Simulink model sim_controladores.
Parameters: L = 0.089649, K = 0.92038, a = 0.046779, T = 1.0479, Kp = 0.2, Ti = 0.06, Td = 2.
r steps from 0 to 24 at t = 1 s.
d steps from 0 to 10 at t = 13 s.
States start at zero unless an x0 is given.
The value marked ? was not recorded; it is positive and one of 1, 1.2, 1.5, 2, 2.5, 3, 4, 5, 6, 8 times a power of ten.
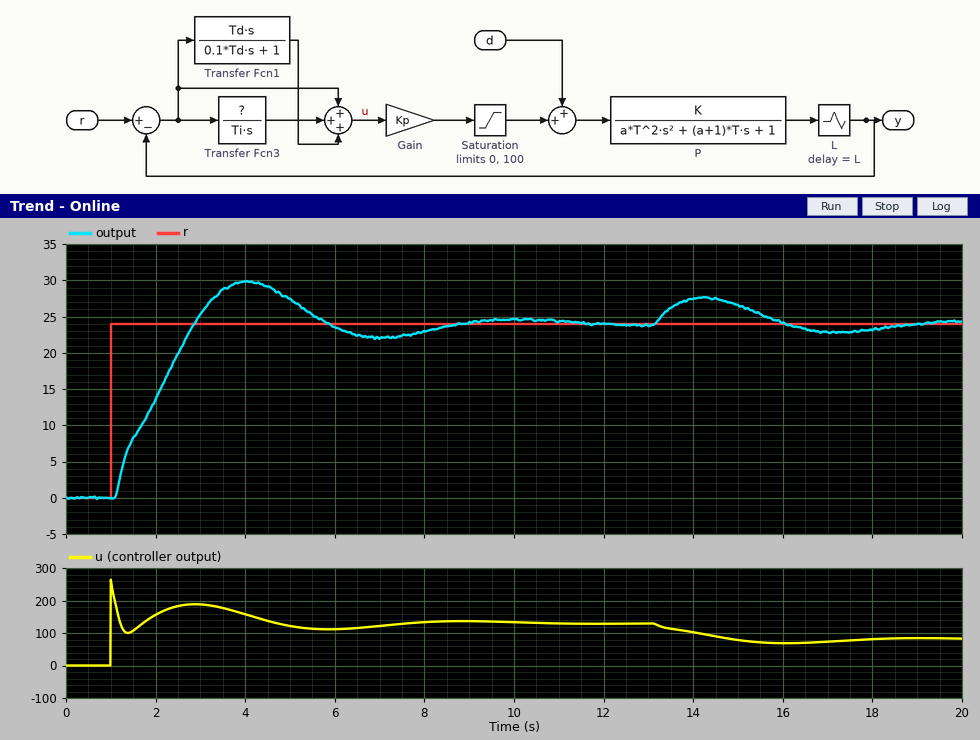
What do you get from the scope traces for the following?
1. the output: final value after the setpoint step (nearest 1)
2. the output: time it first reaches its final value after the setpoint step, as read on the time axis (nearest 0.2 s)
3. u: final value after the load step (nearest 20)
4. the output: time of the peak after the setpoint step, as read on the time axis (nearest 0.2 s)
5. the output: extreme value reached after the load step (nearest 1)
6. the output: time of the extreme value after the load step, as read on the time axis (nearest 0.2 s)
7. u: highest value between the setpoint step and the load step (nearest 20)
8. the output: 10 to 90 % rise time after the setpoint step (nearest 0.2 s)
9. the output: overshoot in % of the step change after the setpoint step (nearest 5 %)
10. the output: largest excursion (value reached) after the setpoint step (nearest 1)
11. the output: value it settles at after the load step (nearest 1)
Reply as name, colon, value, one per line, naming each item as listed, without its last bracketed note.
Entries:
the output: final value after the setpoint step: 24
the output: time it first reaches its final value after the setpoint step, as read on the time axis: 2.8 s
u: final value after the load step: 80
the output: time of the peak after the setpoint step, as read on the time axis: 4.0 s
the output: extreme value reached after the load step: 28
the output: time of the extreme value after the load step, as read on the time axis: 14.2 s
u: highest value between the setpoint step and the load step: 260
the output: 10 to 90 % rise time after the setpoint step: 1.4 s
the output: overshoot in % of the step change after the setpoint step: 25 %
the output: largest excursion (value reached) after the setpoint step: 30
the output: value it settles at after the load step: 24
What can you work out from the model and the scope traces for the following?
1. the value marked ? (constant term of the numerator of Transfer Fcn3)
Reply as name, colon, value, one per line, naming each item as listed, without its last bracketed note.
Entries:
the value marked ?: 0.6
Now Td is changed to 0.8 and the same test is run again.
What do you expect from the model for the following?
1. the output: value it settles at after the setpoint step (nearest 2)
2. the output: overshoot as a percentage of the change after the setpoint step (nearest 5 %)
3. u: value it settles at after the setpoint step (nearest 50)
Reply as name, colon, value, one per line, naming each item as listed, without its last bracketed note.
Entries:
the output: value it settles at after the setpoint step: 24
the output: overshoot as a percentage of the change after the setpoint step: 30 %
u: value it settles at after the setpoint step: 150
